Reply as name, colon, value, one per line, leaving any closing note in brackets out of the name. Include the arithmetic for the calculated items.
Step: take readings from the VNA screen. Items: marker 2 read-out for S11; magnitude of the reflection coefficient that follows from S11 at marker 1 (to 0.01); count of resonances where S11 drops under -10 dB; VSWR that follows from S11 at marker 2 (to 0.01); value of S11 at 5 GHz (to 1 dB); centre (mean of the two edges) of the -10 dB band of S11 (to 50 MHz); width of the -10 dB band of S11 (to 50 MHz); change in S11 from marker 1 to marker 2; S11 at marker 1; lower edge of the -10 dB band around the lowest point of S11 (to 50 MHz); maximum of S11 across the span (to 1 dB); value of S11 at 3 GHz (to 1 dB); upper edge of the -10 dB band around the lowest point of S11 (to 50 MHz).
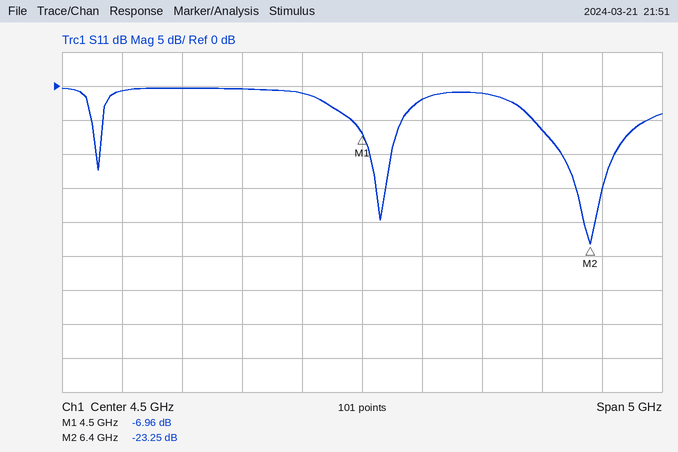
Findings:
marker 2 read-out for S11: -23.25 dB
magnitude of the reflection coefficient that follows from S11 at marker 1: 10^(-6.96/20) ≈ 0.45
count of resonances where S11 drops under -10 dB: 3
VSWR that follows from S11 at marker 2: (1 + 0.0688)/(1 − 0.0688) ≈ 1.15
value of S11 at 5 GHz: -2 dB
centre (mean of the two edges) of the -10 dB band of S11: 6.40 GHz
width of the -10 dB band of S11: 6.60 GHz − 6.15 GHz = 450 MHz
change in S11 from marker 1 to marker 2: -23.25 − (-6.96) = -16.29 dB
S11 at marker 1: -6.96 dB
lower edge of the -10 dB band around the lowest point of S11: 6.15 GHz
maximum of S11 across the span: 0 dB
value of S11 at 3 GHz: 0 dB
upper edge of the -10 dB band around the lowest point of S11: 6.60 GHz
